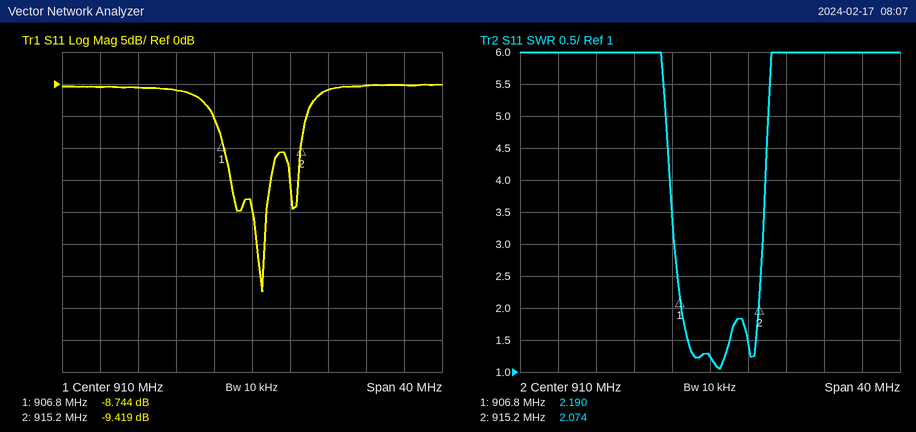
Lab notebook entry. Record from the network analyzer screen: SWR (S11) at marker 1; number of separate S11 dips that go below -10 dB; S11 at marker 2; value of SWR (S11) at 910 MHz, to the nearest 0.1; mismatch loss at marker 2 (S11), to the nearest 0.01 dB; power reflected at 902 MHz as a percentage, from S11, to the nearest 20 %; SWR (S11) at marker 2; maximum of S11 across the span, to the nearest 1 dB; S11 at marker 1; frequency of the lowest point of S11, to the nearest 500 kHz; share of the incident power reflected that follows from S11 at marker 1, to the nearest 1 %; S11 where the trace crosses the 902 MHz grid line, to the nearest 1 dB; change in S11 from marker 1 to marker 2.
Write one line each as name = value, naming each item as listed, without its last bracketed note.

SWR (S11) at marker 1 = 2.190
number of separate S11 dips that go below -10 dB = 2
S11 at marker 2 = -9.419 dB
value of SWR (S11) at 910 MHz, to the nearest 0.1 = 1.2
mismatch loss at marker 2 (S11), to the nearest 0.01 dB = 0.53 dB
power reflected at 902 MHz as a percentage, from S11, to the nearest 20 % = 80 %
SWR (S11) at marker 2 = 2.074
maximum of S11 across the span, to the nearest 1 dB = 0 dB
S11 at marker 1 = -8.744 dB
frequency of the lowest point of S11, to the nearest 500 kHz = 911.0 MHz
share of the incident power reflected that follows from S11 at marker 1, to the nearest 1 % = 13 %
S11 where the trace crosses the 902 MHz grid line, to the nearest 1 dB = -1 dB
change in S11 from marker 1 to marker 2 = -0.675 dB
